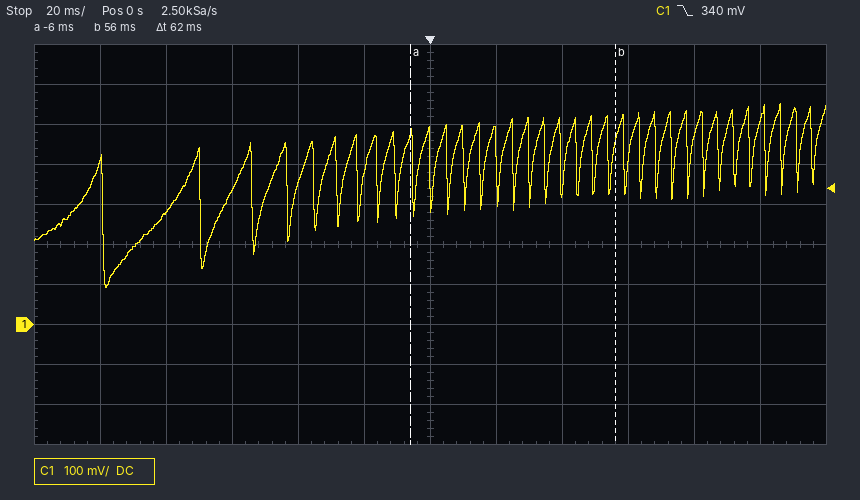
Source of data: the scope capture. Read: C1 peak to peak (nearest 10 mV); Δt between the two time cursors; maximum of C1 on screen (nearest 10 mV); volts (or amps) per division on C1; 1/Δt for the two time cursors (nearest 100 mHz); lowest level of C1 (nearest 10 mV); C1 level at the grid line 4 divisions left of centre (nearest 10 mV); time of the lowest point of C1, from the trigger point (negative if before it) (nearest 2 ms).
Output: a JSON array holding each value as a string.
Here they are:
["460 mV", "62 ms", "550 mV", "100 mV", "16.1 Hz", "90 mV", "280 mV", "-98 ms"]
